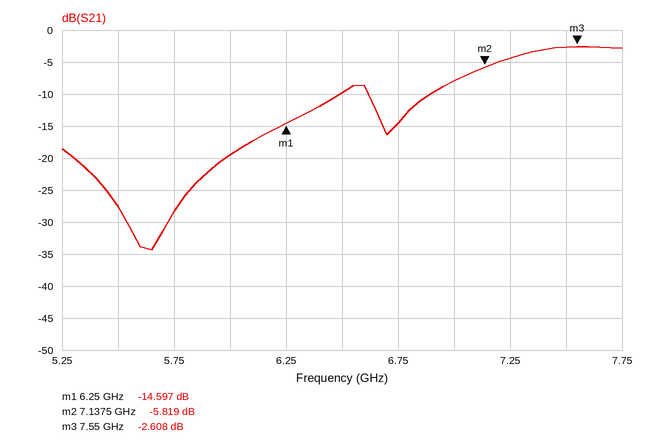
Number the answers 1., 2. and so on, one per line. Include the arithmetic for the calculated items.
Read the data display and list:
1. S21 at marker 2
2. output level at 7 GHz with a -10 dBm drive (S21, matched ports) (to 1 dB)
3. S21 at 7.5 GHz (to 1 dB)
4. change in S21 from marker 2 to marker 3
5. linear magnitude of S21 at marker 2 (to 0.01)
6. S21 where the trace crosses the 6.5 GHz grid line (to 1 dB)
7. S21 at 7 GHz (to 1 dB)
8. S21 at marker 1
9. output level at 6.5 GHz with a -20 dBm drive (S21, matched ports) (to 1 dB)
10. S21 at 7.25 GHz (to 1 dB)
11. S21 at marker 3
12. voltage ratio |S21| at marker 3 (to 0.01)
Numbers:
1. -5.819 dB
2. -10 dBm + (-8 dB) = -18 dBm
3. -3 dB
4. -2.608 − (-5.819) = 3.211 dB
5. 10^(-5.819/20) ≈ 0.51
6. -10 dB
7. -8 dB
8. -14.597 dB
9. -20 dBm + (-10 dB) = -30 dBm
10. -4 dB
11. -2.608 dB
12. 10^(-2.608/20) ≈ 0.74
